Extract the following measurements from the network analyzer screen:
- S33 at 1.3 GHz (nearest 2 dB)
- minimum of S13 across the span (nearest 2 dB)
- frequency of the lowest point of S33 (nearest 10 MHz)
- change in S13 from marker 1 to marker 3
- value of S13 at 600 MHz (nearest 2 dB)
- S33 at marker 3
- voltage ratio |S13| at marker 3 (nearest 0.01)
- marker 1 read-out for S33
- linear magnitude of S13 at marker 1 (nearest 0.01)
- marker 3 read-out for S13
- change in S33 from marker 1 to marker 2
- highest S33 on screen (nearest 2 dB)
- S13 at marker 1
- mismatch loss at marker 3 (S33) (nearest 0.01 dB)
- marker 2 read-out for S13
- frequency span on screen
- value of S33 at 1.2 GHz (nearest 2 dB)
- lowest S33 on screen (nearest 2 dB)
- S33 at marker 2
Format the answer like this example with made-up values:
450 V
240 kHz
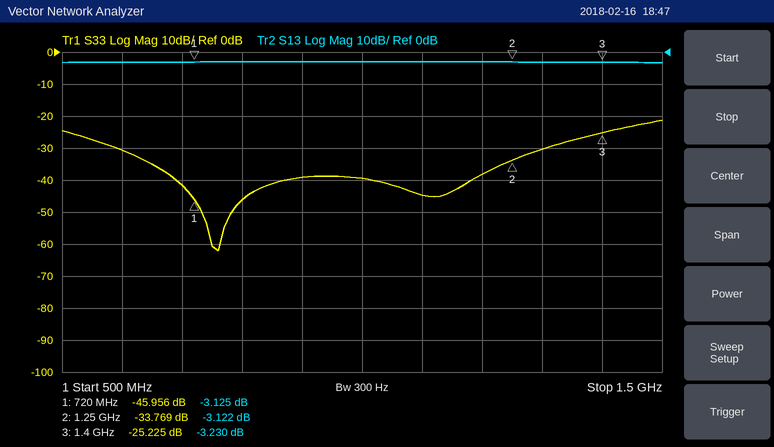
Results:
-30 dB
-4 dB
760 MHz
-0.105 dB
-4 dB
-25.225 dB
0.69
-45.956 dB
0.70
-3.230 dB
12.187 dB
-22 dB
-3.125 dB
0.01 dB
-3.122 dB
1 GHz
-38 dB
-62 dB
-33.769 dB
